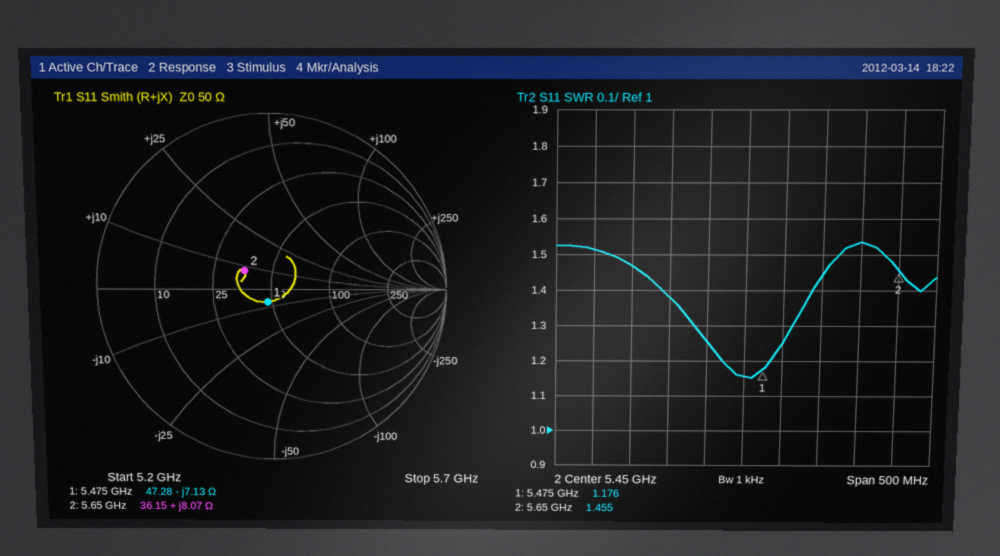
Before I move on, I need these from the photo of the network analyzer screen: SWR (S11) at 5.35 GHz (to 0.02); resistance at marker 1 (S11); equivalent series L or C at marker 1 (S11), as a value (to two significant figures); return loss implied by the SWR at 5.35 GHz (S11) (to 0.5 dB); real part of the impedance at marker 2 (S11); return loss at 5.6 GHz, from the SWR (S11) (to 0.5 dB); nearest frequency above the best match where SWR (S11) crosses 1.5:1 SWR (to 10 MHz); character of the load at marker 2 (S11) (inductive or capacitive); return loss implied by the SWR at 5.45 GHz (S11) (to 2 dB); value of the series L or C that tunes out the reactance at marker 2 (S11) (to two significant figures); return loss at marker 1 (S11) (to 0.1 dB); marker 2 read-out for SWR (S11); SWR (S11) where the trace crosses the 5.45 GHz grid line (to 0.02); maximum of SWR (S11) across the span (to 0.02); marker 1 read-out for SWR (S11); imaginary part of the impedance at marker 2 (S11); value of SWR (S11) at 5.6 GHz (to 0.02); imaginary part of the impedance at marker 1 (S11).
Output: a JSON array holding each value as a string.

["1.38", "47.28 Ω", "4.1 pF", "16.0 dB", "36.15 Ω", "13.5 dB", "5.57 GHz", "inductive", "22 dB", "3.5 pF", "22.1 dB", "1.455", "1.16", "1.54", "1.176", "+8.07 Ω", "1.54", "-7.13 Ω"]
